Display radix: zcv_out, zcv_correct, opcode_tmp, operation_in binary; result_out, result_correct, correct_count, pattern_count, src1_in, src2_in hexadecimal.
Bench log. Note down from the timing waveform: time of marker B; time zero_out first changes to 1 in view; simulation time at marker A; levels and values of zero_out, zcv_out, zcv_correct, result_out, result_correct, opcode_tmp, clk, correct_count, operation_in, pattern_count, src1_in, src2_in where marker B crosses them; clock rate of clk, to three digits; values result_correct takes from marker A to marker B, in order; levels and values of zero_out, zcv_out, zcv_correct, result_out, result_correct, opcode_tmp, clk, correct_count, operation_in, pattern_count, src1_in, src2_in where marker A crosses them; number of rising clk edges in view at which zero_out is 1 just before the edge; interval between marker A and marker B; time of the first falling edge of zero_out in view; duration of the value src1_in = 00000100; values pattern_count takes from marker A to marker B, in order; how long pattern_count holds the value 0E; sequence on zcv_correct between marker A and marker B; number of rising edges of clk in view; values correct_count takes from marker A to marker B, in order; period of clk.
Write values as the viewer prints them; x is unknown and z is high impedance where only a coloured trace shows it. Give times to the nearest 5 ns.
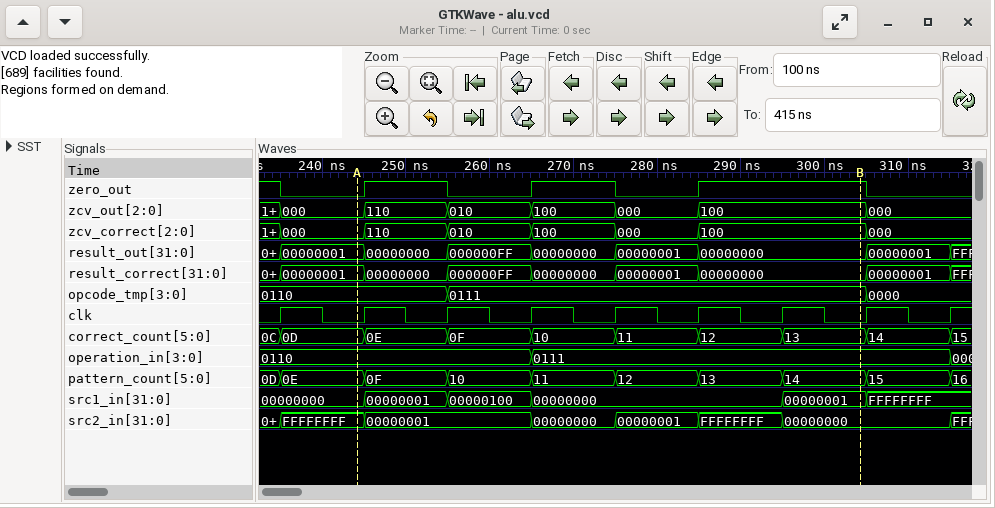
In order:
305 ns
245 ns
245 ns
zero_out=1, zcv_out=100, zcv_correct=100, result_out=00000000, result_correct=00000000, opcode_tmp=0111, clk=0, correct_count=13, operation_in=0111, pattern_count=14, src1_in=00000001, src2_in=00000000
100 MHz
00000001, 00000000, 000000FF, 00000000, 00000001, 00000000
zero_out=0, zcv_out=000, zcv_correct=000, result_out=00000001, result_correct=00000001, opcode_tmp=0110, clk=0, correct_count=0D, operation_in=0110, pattern_count=0E, src1_in=00000000, src2_in=FFFFFFFF
5
60 ns
235 ns
10 ns
0E, 0F, 10, 11, 12, 13, 14
10 ns
000, 110, 010, 100, 000, 100
9
0D, 0E, 0F, 10, 11, 12, 13
10 ns
